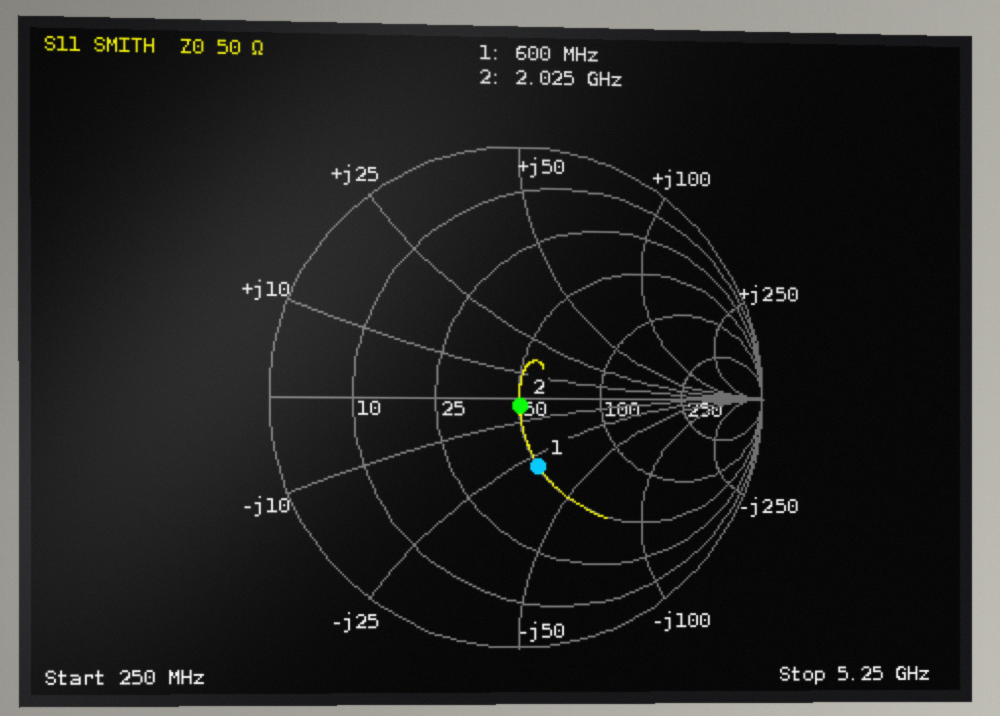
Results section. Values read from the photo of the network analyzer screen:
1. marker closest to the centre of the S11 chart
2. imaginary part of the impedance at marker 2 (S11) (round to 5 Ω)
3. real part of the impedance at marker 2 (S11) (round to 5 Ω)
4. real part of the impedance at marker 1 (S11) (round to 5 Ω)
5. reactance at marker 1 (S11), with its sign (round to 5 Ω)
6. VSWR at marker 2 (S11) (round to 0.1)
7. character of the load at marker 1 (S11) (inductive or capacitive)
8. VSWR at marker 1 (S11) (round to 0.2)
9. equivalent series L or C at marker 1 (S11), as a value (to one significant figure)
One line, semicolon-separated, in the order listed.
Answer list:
marker 2; -5 Ω; 50 Ω; 50 Ω; -30 Ω; 1.1; capacitive; 1.8; 9 pF
